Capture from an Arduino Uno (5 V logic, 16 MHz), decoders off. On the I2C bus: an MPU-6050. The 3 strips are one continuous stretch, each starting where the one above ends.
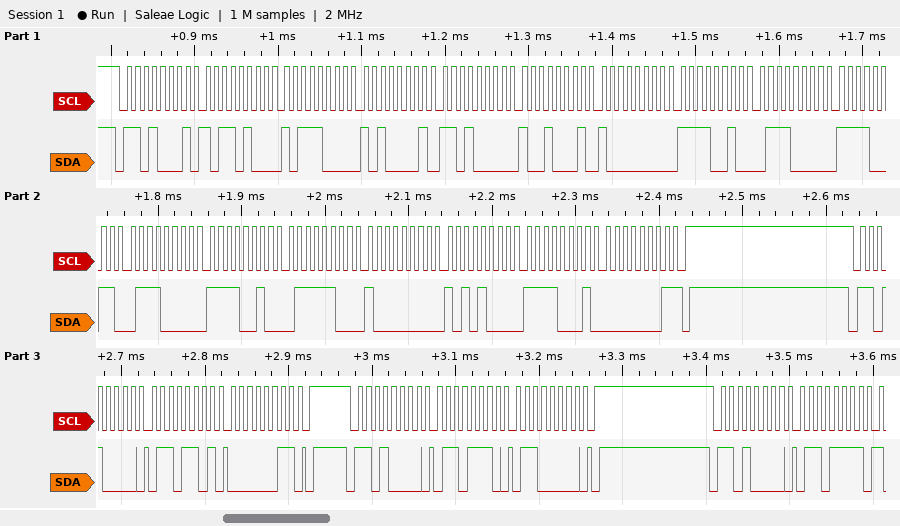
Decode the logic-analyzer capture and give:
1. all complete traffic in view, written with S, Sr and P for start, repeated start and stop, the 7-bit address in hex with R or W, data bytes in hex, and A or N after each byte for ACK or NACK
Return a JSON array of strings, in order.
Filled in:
["S 68R A B4 A B8 A A1 A D0 A 91 A 80 A F2 A 70 A F3 A 70 A F2 A 7C A 80 A A8 A F1 A 01 N P S 68W A 6D A 03 A P S 68W A 6E A 60 A P S 68W A 6F A"]
